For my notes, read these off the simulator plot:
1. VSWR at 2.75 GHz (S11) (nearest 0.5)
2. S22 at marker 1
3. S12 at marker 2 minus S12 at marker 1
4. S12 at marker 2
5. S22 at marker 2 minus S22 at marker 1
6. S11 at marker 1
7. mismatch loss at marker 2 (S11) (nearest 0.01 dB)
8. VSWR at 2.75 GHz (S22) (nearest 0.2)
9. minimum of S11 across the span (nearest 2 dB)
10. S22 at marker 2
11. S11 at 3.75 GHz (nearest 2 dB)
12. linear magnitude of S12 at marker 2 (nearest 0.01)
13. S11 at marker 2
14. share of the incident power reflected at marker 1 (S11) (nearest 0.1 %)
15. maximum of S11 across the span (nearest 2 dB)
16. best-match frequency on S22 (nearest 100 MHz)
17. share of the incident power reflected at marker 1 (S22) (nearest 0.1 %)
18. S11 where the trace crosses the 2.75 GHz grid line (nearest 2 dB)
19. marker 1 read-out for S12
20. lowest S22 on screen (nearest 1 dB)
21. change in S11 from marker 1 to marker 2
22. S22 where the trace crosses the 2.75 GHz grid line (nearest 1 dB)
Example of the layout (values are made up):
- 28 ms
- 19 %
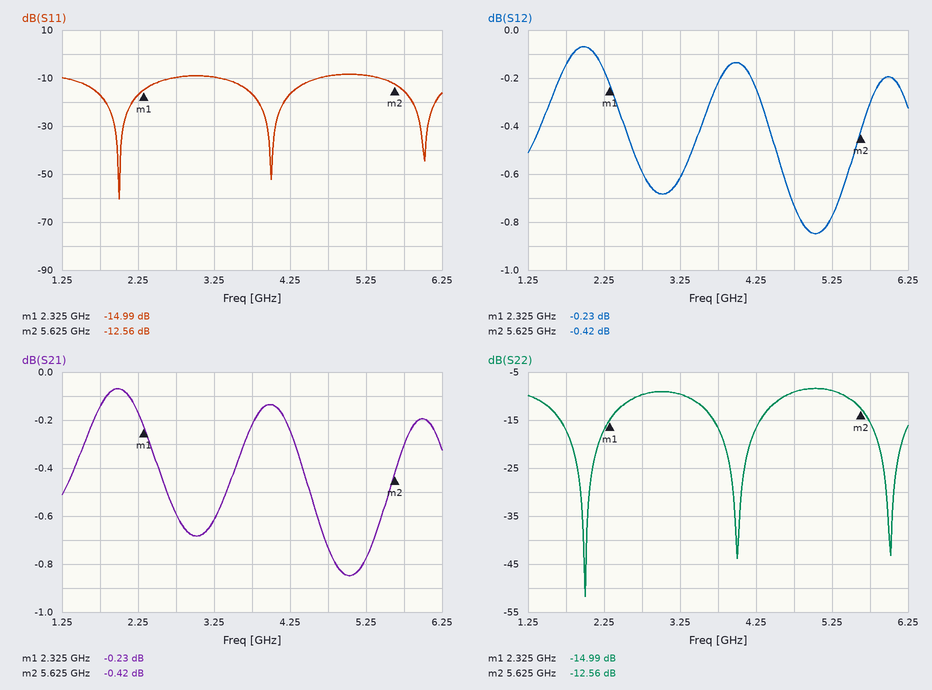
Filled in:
- 2.0
- -14.99 dB
- -0.19 dB
- -0.42 dB
- 2.43 dB
- -14.99 dB
- 0.25 dB
- 2.0
- -60 dB
- -12.56 dB
- -16 dB
- 0.95
- -12.56 dB
- 3.2 %
- -8 dB
- 2.0 GHz
- 3.2 %
- -10 dB
- -0.23 dB
- -52 dB
- 2.43 dB
- -10 dB
